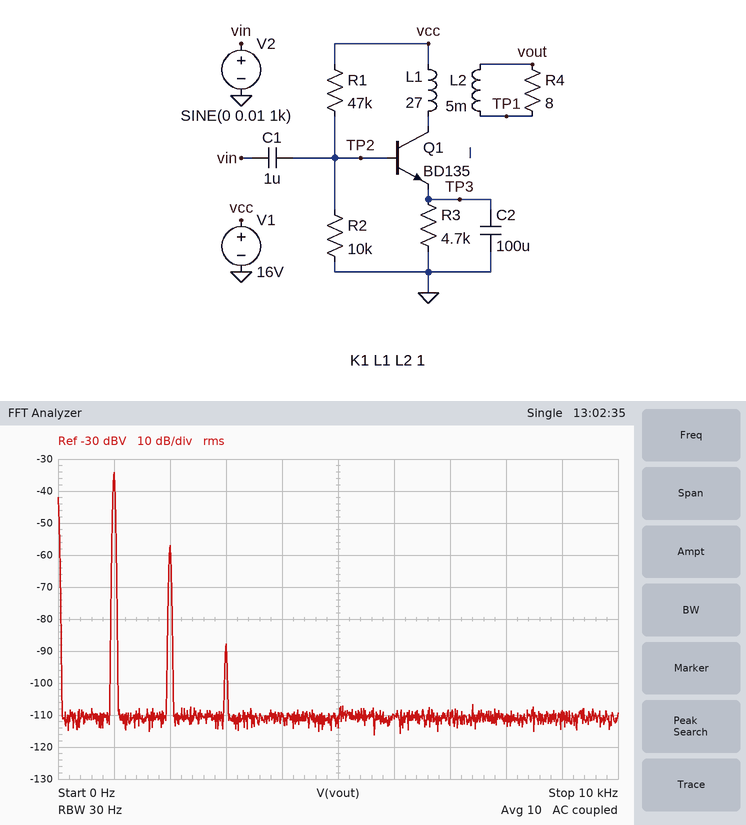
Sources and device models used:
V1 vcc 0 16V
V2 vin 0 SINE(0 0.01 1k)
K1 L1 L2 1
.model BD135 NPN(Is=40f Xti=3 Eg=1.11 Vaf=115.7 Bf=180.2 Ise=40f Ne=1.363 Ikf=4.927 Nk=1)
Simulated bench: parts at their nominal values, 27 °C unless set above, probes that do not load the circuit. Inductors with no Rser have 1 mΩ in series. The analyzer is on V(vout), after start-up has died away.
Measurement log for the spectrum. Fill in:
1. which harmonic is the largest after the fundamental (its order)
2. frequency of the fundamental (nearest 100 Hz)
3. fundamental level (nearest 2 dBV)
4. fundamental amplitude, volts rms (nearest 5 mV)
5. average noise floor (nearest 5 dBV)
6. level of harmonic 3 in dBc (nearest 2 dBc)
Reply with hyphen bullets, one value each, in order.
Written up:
- 2
- 1.0 kHz
- -34 dBV
- 20 mV
- -110 dBV
- -54 dBc
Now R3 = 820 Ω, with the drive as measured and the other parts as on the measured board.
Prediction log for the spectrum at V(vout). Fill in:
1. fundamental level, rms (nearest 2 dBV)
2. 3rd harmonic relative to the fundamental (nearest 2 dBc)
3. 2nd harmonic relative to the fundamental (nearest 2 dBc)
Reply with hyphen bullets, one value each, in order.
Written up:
- -26 dBV
- -24 dBc
- -18 dBc
